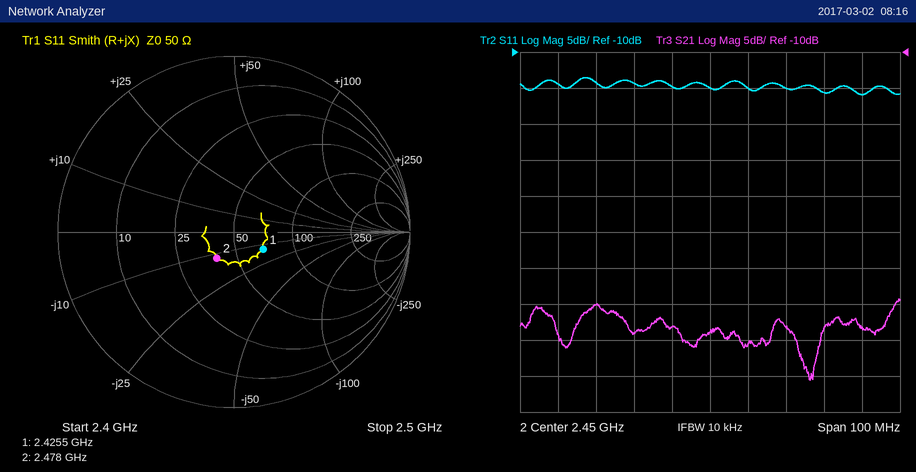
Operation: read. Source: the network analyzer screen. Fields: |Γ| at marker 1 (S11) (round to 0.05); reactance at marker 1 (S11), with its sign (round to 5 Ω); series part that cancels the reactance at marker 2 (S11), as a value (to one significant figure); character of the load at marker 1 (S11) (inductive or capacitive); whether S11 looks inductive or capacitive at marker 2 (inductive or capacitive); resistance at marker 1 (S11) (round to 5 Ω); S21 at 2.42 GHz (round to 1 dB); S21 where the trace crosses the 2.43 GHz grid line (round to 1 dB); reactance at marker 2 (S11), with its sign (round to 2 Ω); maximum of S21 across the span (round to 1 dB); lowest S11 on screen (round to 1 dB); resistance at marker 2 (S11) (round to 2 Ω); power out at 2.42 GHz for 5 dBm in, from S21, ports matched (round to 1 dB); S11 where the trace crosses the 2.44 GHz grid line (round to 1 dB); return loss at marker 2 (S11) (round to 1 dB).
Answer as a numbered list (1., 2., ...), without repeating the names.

1. 0.20
2. -15 Ω
3. 800 pH
4. capacitive
5. capacitive
6. 70 Ω
7. -45 dB
8. -49 dB
9. -12 Ω
10. -44 dB
11. -16 dB
12. 40 Ω
13. -40 dBm
14. -15 dB
15. 15 dB
